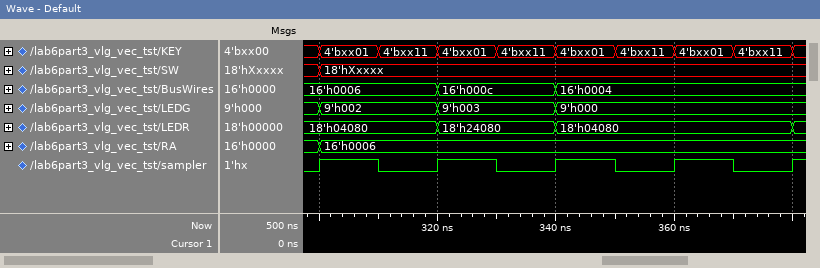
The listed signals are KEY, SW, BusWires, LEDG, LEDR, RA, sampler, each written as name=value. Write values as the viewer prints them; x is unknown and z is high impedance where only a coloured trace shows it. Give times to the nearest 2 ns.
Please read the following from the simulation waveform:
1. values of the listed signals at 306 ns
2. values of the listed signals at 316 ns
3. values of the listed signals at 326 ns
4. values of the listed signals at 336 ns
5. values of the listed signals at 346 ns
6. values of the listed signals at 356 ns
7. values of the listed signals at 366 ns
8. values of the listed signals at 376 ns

KEY=4'bxx01, SW=18'hXxxxx, BusWires=16'h0006, LEDG=9'h002, LEDR=18'h04080, RA=16'h0006, sampler=1
KEY=4'bxx11, SW=18'hXxxxx, BusWires=16'h0006, LEDG=9'h002, LEDR=18'h04080, RA=16'h0006, sampler=0
KEY=4'bxx01, SW=18'hXxxxx, BusWires=16'h000c, LEDG=9'h003, LEDR=18'h24080, RA=16'h0006, sampler=1
KEY=4'bxx11, SW=18'hXxxxx, BusWires=16'h000c, LEDG=9'h003, LEDR=18'h24080, RA=16'h0006, sampler=0
KEY=4'bxx01, SW=18'hXxxxx, BusWires=16'h0004, LEDG=9'h000, LEDR=18'h04080, RA=16'h0006, sampler=1
KEY=4'bxx11, SW=18'hXxxxx, BusWires=16'h0004, LEDG=9'h000, LEDR=18'h04080, RA=16'h0006, sampler=0
KEY=4'bxx01, SW=18'hXxxxx, BusWires=16'h0004, LEDG=9'h000, LEDR=18'h04080, RA=16'h0006, sampler=1
KEY=4'bxx11, SW=18'hXxxxx, BusWires=16'h0004, LEDG=9'h000, LEDR=18'h04080, RA=16'h0006, sampler=0
